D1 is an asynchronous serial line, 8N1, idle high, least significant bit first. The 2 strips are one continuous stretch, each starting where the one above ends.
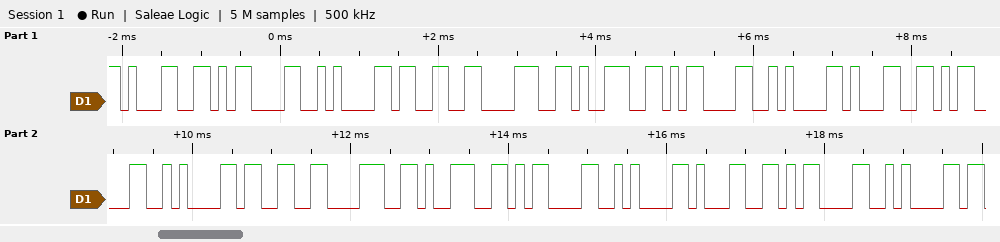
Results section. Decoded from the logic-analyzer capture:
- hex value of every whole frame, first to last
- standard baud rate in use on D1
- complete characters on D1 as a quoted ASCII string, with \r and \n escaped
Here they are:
31 0D 0A 33 38 39 0D 0A 31 0D 0A 33 38 39 0D 0A 31 0D 0A
9600 baud
"1\r\n389\r\n1\r\n389\r\n1\r\n"
